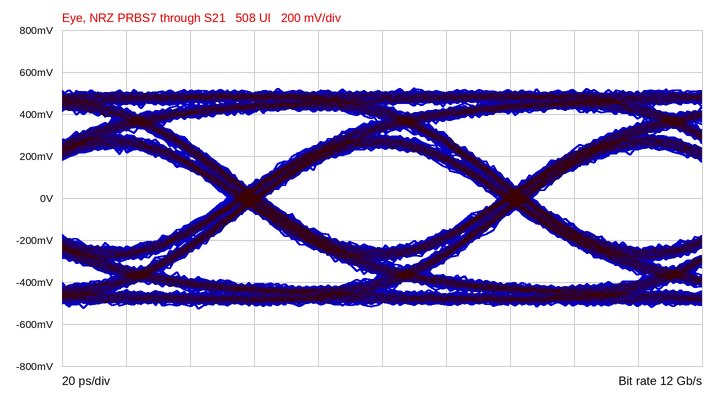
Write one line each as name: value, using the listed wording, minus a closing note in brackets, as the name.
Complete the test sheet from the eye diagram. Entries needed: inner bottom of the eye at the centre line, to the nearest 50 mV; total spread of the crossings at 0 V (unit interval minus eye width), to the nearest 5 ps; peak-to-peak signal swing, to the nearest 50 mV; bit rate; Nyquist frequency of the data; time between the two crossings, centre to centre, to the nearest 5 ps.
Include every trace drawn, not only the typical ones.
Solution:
inner bottom of the eye at the centre line, to the nearest 50 mV: -250 mV
total spread of the crossings at 0 V (unit interval minus eye width), to the nearest 5 ps: 10 ps
peak-to-peak signal swing, to the nearest 50 mV: 1.05 V
bit rate: 12 Gb/s
Nyquist frequency of the data: 6 GHz
time between the two crossings, centre to centre, to the nearest 5 ps: 85 ps
